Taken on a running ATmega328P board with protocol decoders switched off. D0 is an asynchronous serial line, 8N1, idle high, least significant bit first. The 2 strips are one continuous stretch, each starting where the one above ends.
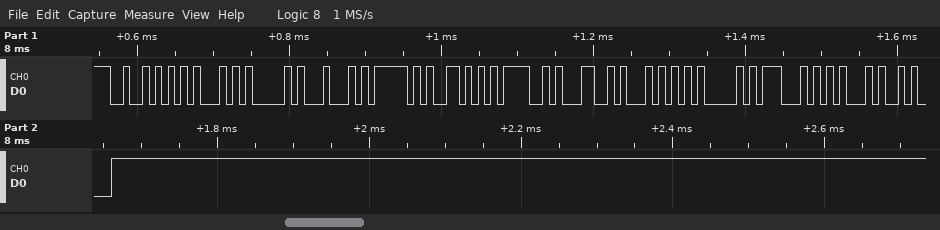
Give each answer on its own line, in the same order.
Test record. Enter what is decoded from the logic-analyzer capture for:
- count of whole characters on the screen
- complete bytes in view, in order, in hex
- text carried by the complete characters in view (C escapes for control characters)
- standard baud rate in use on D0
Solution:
13
52 45 41 44 5F 56 4F 4C 54 41 47 45 0A
"READ_VOLTAGE\n"
115200 baud
